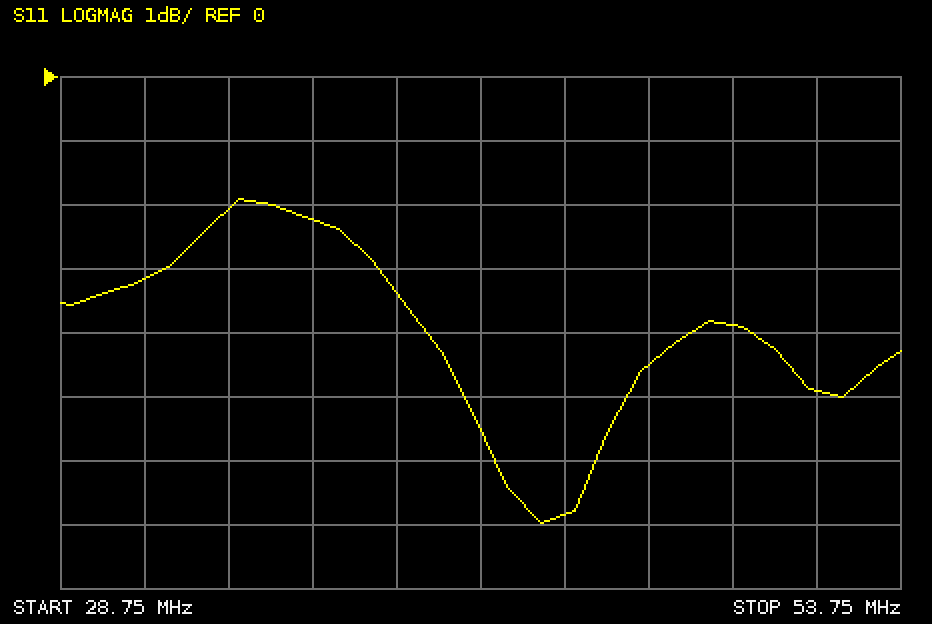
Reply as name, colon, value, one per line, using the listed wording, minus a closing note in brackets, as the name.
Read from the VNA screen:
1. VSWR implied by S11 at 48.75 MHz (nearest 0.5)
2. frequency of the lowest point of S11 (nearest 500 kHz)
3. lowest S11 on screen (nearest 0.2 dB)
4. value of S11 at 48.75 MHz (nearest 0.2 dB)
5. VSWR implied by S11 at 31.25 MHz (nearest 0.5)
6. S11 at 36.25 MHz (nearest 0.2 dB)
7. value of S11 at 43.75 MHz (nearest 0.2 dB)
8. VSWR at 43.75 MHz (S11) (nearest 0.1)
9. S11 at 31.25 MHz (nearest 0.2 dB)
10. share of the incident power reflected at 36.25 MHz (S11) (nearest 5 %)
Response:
VSWR implied by S11 at 48.75 MHz: 4.5
frequency of the lowest point of S11: 43.0 MHz
lowest S11 on screen: -7.0 dB
value of S11 at 48.75 MHz: -3.8 dB
VSWR implied by S11 at 31.25 MHz: 5.5
S11 at 36.25 MHz: -2.2 dB
value of S11 at 43.75 MHz: -6.8 dB
VSWR at 43.75 MHz (S11): 2.7
S11 at 31.25 MHz: -3.2 dB
share of the incident power reflected at 36.25 MHz (S11): 60 %
